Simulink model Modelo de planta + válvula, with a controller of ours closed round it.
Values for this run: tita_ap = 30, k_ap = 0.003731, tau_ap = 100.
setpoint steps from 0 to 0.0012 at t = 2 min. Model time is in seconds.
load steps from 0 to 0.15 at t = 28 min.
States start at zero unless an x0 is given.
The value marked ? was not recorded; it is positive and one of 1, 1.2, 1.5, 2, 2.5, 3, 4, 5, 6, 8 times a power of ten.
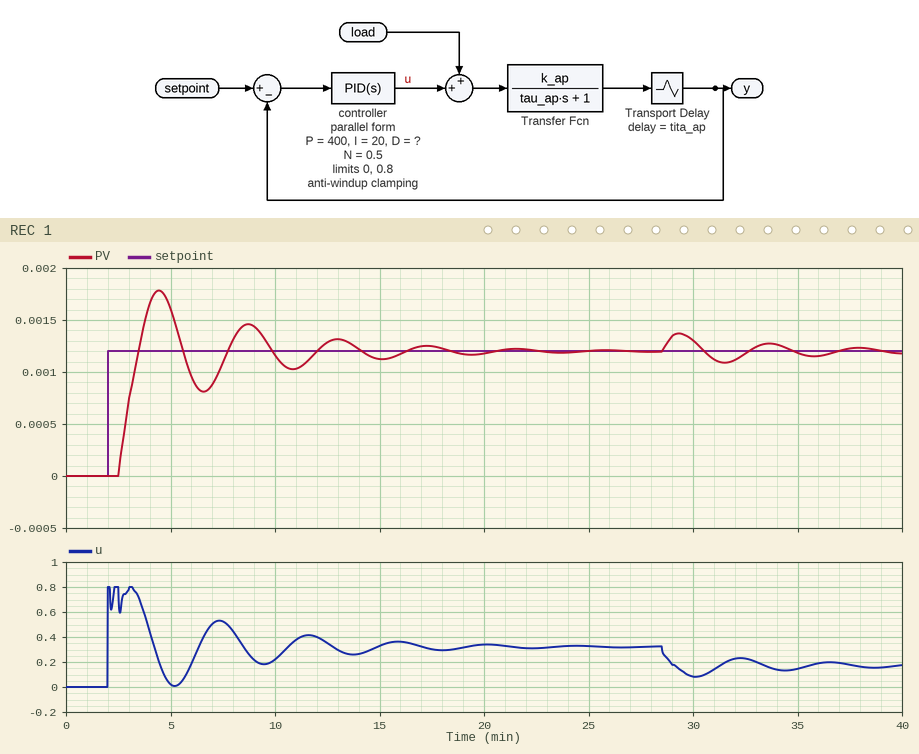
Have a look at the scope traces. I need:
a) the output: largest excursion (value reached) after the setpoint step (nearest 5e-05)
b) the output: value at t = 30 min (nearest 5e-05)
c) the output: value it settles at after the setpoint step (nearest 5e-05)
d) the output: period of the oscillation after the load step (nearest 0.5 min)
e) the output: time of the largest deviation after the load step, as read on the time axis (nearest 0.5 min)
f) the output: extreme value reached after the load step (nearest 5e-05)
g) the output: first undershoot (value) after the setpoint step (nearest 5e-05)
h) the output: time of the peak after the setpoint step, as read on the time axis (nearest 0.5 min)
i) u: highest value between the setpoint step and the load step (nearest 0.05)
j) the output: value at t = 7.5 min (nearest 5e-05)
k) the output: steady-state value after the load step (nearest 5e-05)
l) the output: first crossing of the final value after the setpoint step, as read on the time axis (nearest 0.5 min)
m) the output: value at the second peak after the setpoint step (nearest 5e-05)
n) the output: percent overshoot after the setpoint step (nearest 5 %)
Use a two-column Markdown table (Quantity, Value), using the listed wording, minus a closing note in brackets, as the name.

| Quantity | Value |
|---|---|
| the output: largest excursion (value reached) after the setpoint step | 0.00180 |
| the output: value at t = 30 min | 0.00130 |
| the output: value it settles at after the setpoint step | 0.00120 |
| the output: period of the oscillation after the load step | 4.5 min |
| the output: time of the largest deviation after the load step, as read on the time axis | 29.5 min |
| the output: extreme value reached after the load step | 0.00135 |
| the output: first undershoot (value) after the setpoint step | 0.00080 |
| the output: time of the peak after the setpoint step, as read on the time axis | 4.5 min |
| u: highest value between the setpoint step and the load step | 0.80 |
| the output: value at t = 7.5 min | 0.00110 |
| the output: steady-state value after the load step | 0.00120 |
| the output: first crossing of the final value after the setpoint step, as read on the time axis | 3.5 min |
| the output: value at the second peak after the setpoint step | 0.00145 |
| the output: percent overshoot after the setpoint step | 50 % |
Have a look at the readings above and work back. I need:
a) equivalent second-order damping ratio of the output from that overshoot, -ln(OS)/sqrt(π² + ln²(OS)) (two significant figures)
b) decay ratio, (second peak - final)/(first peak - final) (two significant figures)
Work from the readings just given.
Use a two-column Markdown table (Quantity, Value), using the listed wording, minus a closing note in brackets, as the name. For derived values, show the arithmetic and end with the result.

| Quantity | Value |
|---|---|
| equivalent second-order damping ratio of the output from that overshoot, -ln(OS)/sqrt(π² + ln²(OS)) | ln(0.5) = -0.693; 0.693 / sqrt(9.870 + 0.480) = 0.22 |
| decay ratio, (second peak - final)/(first peak - final) | (0.00145 - 0.0012) / (0.0018 - 0.0012) = 0.42 |
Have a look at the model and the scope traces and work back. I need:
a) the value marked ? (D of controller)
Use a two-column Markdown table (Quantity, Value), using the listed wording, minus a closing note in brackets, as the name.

| Quantity | Value |
|---|---|
| the value marked ? | 10000 |
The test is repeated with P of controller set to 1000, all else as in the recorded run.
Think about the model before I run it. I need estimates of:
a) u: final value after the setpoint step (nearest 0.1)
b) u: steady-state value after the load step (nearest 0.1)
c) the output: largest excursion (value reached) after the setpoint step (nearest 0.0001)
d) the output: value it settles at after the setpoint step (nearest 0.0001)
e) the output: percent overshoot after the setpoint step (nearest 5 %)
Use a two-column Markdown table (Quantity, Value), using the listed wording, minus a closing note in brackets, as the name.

| Quantity | Value |
|---|---|
| u: final value after the setpoint step | 0.3 |
| u: steady-state value after the load step | 0.2 |
| the output: largest excursion (value reached) after the setpoint step | 0.0013 |
| the output: value it settles at after the setpoint step | 0.0012 |
| the output: percent overshoot after the setpoint step | 10 % |
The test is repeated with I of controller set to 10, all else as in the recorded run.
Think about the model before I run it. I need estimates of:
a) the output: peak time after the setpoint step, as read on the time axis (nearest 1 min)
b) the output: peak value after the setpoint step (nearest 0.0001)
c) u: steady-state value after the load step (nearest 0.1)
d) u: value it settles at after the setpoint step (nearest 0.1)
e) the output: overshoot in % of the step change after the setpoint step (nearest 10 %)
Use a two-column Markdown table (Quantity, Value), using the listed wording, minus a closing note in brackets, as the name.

| Quantity | Value |
|---|---|
| the output: peak time after the setpoint step, as read on the time axis | 5 min |
| the output: peak value after the setpoint step | 0.0016 |
| u: steady-state value after the load step | 0.2 |
| u: value it settles at after the setpoint step | 0.3 |
| the output: overshoot in % of the step change after the setpoint step | 30 % |
